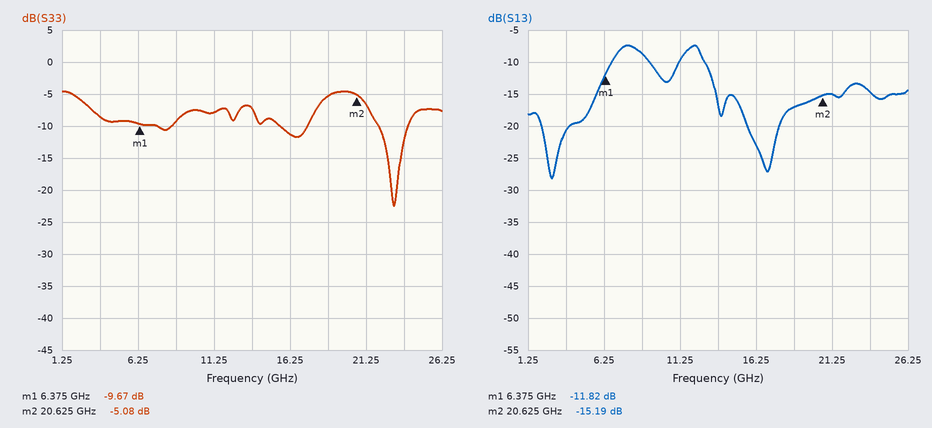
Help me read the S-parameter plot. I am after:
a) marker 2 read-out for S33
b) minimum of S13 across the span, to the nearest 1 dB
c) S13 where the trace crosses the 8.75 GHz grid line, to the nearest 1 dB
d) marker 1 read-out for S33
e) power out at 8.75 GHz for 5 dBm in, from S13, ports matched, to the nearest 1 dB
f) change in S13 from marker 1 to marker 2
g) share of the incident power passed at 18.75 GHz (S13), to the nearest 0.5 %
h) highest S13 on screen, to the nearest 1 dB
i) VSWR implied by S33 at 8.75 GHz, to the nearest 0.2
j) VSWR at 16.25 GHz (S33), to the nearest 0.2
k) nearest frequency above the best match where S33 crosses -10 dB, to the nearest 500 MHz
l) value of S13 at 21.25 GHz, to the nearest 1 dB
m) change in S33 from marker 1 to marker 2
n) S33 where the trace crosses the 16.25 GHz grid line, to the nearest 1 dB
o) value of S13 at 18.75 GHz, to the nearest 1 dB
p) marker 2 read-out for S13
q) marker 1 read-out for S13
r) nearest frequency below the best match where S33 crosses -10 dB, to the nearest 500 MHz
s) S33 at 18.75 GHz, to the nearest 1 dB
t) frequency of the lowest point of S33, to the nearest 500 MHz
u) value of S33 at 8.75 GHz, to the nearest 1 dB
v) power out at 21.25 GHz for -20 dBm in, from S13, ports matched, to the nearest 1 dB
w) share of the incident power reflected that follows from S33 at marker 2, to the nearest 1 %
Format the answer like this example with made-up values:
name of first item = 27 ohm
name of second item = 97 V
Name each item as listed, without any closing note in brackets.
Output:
marker 2 read-out for S33 = -5.08 dB
minimum of S13 across the span, to the nearest 1 dB = -28 dB
S13 where the trace crosses the 8.75 GHz grid line, to the nearest 1 dB = -9 dB
marker 1 read-out for S33 = -9.67 dB
power out at 8.75 GHz for 5 dBm in, from S13, ports matched, to the nearest 1 dB = -4 dBm
change in S13 from marker 1 to marker 2 = -3.37 dB
share of the incident power passed at 18.75 GHz (S13), to the nearest 0.5 % = 2.0 %
highest S13 on screen, to the nearest 1 dB = -7 dB
VSWR implied by S33 at 8.75 GHz, to the nearest 0.2 = 2.0
VSWR at 16.25 GHz (S33), to the nearest 0.2 = 1.8
nearest frequency above the best match where S33 crosses -10 dB, to the nearest 500 MHz = 24.0 GHz
value of S13 at 21.25 GHz, to the nearest 1 dB = -15 dB
change in S33 from marker 1 to marker 2 = 4.59 dB
S33 where the trace crosses the 16.25 GHz grid line, to the nearest 1 dB = -11 dB
value of S13 at 18.75 GHz, to the nearest 1 dB = -17 dB
marker 2 read-out for S13 = -15.19 dB
marker 1 read-out for S13 = -11.82 dB
nearest frequency below the best match where S33 crosses -10 dB, to the nearest 500 MHz = 22.0 GHz
S33 at 18.75 GHz, to the nearest 1 dB = -5 dB
frequency of the lowest point of S33, to the nearest 500 MHz = 23.0 GHz
value of S33 at 8.75 GHz, to the nearest 1 dB = -9 dB
power out at 21.25 GHz for -20 dBm in, from S13, ports matched, to the nearest 1 dB = -35 dBm
share of the incident power reflected that follows from S33 at marker 2, to the nearest 1 % = 31 %
